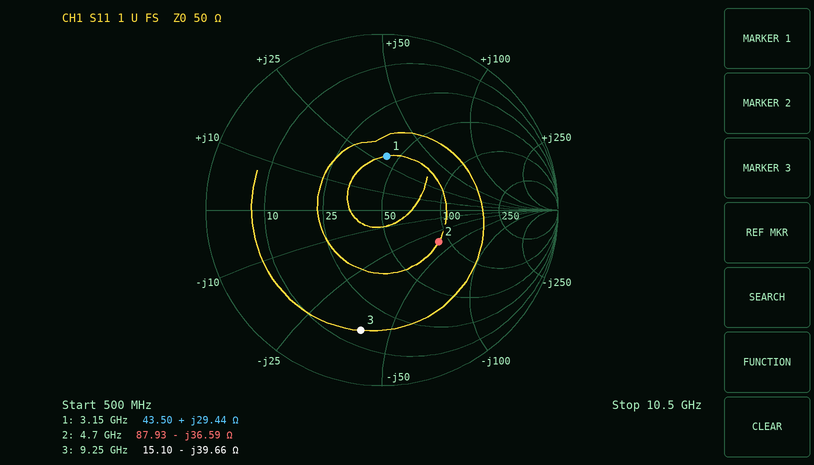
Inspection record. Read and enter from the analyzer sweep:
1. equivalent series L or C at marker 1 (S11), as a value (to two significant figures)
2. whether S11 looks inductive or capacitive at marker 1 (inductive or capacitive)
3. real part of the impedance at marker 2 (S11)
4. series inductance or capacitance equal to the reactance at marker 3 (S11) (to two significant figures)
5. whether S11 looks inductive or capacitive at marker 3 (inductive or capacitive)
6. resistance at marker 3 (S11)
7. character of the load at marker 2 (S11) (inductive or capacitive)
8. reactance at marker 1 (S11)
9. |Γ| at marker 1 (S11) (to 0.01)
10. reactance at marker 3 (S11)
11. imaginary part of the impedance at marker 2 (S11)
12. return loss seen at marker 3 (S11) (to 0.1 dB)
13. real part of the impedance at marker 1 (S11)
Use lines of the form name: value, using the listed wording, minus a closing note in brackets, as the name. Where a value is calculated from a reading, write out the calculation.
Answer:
equivalent series L or C at marker 1 (S11), as a value: L = 29.44 Ω/(2π × 3.15 GHz) ≈ 1.5 nH
whether S11 looks inductive or capacitive at marker 1: inductive
real part of the impedance at marker 2: 87.93 Ω
series inductance or capacitance equal to the reactance at marker 3 (S11): C = 1/(2π × 9.25 GHz × 39.66 Ω) ≈ 434 fF, so 430 fF to two significant figures
whether S11 looks inductive or capacitive at marker 3: capacitive
resistance at marker 3: 15.10 Ω
character of the load at marker 2 (S11): capacitive
reactance at marker 1: +29.44 Ω
|Γ| at marker 1 (S11): 0.31
reactance at marker 3: -39.66 Ω
imaginary part of the impedance at marker 2: -36.59 Ω
return loss seen at marker 3 (S11): 3.2 dB
real part of the impedance at marker 1: 43.50 Ω
